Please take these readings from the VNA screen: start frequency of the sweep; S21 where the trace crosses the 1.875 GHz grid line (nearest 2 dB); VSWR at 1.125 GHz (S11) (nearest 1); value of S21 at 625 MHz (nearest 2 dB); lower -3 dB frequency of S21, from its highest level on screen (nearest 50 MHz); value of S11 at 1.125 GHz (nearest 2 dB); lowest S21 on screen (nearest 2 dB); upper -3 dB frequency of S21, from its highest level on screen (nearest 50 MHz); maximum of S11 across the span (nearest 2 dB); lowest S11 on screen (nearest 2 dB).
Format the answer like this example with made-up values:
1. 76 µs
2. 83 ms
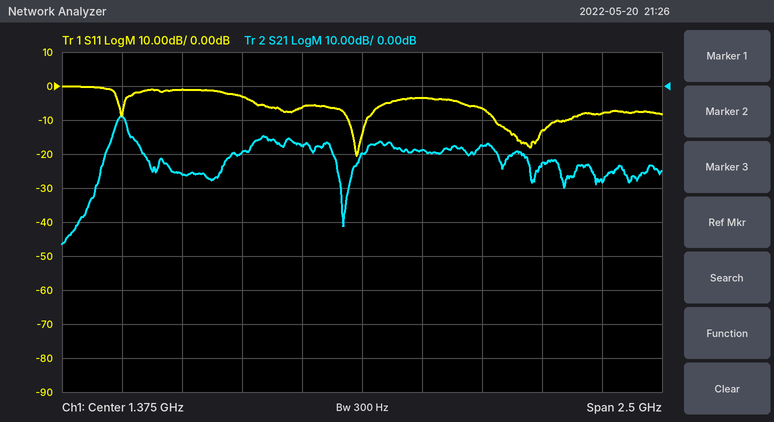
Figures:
1. 125 MHz
2. -18 dB
3. 3
4. -26 dB
5. 350 MHz
6. -6 dB
7. -46 dB
8. 400 MHz
9. 0 dB
10. -20 dB
